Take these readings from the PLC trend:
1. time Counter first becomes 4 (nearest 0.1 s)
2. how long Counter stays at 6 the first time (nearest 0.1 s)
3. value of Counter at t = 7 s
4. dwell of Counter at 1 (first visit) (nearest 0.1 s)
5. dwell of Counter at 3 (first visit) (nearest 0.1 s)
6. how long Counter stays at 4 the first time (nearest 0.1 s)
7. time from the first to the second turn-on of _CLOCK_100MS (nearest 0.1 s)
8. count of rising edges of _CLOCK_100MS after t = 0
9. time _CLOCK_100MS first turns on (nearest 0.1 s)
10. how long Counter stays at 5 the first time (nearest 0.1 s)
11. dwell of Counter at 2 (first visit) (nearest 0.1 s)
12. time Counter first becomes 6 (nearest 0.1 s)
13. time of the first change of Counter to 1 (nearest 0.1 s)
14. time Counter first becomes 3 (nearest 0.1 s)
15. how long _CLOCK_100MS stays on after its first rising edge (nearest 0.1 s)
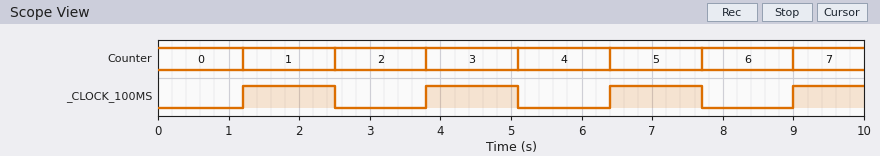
5.1 s
1.3 s
5
1.3 s
1.3 s
1.3 s
2.6 s
4
1.2 s
1.3 s
1.3 s
7.7 s
1.2 s
3.8 s
1.3 s
